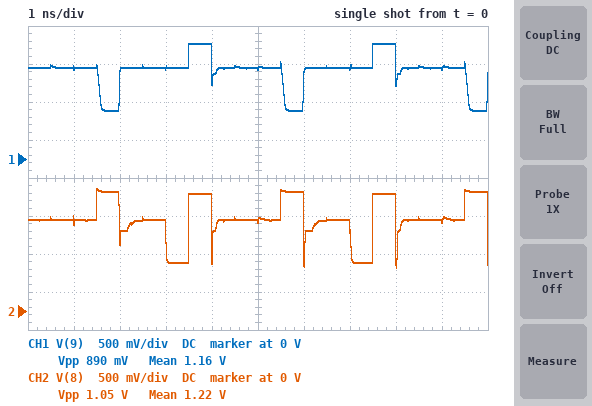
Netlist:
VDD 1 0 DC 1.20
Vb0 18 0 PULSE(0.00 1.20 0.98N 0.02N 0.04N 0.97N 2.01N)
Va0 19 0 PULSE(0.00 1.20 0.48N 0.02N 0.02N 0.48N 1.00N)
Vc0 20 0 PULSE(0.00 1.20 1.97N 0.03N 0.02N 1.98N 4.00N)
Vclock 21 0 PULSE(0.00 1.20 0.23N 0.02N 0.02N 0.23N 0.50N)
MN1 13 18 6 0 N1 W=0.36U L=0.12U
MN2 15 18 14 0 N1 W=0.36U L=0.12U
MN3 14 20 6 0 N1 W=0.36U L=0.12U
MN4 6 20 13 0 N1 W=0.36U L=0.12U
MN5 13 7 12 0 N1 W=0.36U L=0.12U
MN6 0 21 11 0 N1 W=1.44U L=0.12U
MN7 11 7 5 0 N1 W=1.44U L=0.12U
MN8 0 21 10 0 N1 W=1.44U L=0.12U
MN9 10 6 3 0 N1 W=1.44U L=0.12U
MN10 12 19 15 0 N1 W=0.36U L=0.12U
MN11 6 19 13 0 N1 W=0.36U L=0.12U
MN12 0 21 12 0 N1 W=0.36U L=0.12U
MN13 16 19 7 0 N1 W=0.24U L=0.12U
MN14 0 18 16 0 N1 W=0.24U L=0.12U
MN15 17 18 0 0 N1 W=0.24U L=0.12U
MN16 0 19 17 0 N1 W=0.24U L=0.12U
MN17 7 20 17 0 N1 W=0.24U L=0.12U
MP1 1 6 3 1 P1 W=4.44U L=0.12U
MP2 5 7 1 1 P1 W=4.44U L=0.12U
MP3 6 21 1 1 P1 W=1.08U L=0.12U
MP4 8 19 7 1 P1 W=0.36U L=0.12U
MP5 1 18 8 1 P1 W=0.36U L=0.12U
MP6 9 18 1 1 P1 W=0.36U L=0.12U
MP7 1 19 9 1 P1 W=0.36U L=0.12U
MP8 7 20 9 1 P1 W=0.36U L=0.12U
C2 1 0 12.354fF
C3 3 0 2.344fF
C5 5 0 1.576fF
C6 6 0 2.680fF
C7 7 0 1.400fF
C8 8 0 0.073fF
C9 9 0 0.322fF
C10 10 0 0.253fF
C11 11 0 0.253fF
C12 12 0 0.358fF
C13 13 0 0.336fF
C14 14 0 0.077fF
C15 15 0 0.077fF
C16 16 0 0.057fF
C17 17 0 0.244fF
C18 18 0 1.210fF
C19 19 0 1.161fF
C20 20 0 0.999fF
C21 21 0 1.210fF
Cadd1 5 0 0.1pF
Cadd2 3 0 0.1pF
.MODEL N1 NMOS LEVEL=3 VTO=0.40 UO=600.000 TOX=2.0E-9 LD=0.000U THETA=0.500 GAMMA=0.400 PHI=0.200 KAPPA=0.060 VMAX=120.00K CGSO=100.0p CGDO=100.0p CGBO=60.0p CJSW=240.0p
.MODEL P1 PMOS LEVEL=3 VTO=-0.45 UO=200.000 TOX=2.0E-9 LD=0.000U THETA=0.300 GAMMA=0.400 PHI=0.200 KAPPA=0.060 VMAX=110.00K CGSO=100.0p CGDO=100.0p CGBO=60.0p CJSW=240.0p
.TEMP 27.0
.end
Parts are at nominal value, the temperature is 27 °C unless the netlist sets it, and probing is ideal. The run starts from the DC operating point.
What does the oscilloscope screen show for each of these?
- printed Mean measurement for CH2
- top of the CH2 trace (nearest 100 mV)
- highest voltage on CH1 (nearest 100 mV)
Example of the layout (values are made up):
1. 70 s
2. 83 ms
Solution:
1. 1.22 V
2. 1.6 V
3. 1.5 V
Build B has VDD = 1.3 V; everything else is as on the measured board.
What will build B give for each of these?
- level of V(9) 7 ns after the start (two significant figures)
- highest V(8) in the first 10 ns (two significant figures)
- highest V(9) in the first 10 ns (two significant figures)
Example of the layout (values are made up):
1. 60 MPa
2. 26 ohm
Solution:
1. 1.3 V
2. 1.6 V
3. 1.6 V
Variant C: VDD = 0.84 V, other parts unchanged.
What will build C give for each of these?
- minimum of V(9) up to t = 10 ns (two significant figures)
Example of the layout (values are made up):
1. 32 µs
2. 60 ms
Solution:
1. 550 mV
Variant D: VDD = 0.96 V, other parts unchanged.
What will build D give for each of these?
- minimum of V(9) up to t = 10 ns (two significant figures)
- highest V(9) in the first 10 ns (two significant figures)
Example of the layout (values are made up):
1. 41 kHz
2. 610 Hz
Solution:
1. 580 mV
2. 1.4 V
